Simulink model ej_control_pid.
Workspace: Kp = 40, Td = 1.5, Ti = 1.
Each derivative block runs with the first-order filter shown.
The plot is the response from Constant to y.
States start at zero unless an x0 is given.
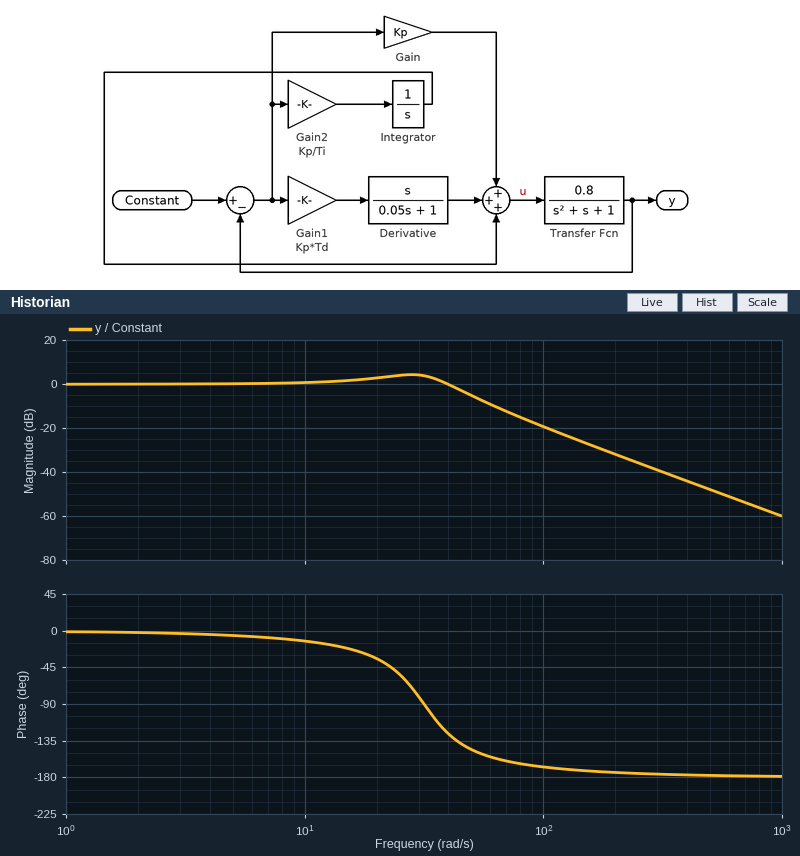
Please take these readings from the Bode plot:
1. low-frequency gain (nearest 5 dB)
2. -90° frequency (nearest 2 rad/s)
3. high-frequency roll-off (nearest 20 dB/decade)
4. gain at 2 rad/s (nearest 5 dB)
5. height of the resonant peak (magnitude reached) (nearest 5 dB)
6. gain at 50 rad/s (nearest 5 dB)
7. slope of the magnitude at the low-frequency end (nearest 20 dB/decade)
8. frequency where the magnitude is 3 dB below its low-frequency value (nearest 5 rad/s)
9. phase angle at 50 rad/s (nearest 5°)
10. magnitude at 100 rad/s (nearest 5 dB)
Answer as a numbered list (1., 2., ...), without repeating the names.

1. 0 dB
2. 32 rad/s
3. -40 dB/decade
4. 0 dB
5. 5 dB
6. -5 dB
7. 0 dB/decade
8. 45 rad/s
9. -145°
10. -20 dB
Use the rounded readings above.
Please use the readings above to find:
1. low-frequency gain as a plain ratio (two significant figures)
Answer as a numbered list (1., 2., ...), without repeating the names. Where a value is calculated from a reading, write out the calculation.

1. 10^(0 / 20) = 1.0
